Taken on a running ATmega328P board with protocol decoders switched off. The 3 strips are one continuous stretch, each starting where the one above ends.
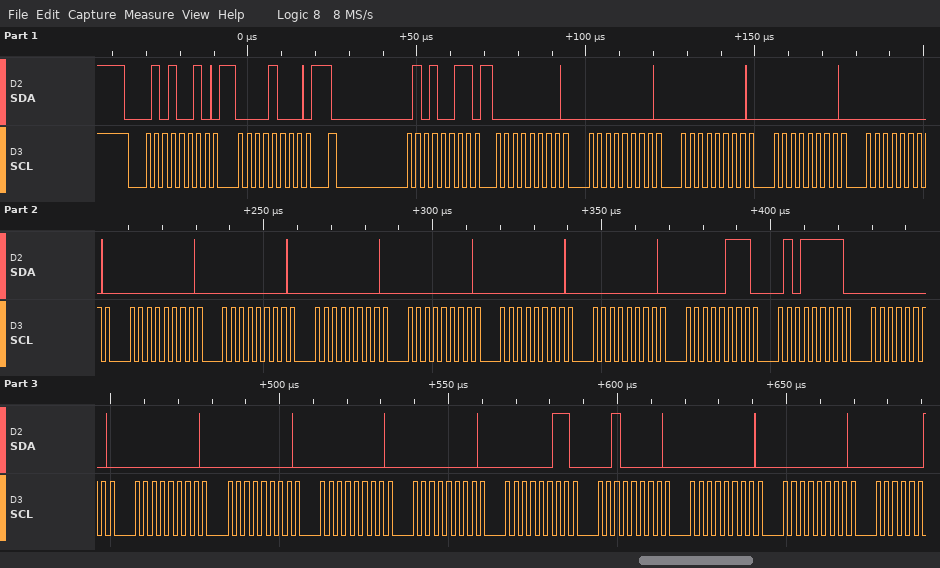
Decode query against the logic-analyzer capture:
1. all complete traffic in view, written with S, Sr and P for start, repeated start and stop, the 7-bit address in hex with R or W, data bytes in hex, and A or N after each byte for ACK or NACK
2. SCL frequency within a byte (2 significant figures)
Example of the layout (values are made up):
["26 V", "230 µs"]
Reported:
["S 29W A 08 A Sr 29R A 00 A 00 A 00 A 00 A 00 A 00 A 00 A 00 A 00 A 00 A 00 A 07 A 5F A 00 A 00 A 00 A 00 A 00 A 03 A 20 A 00 A 00 A", "400 kHz"]
